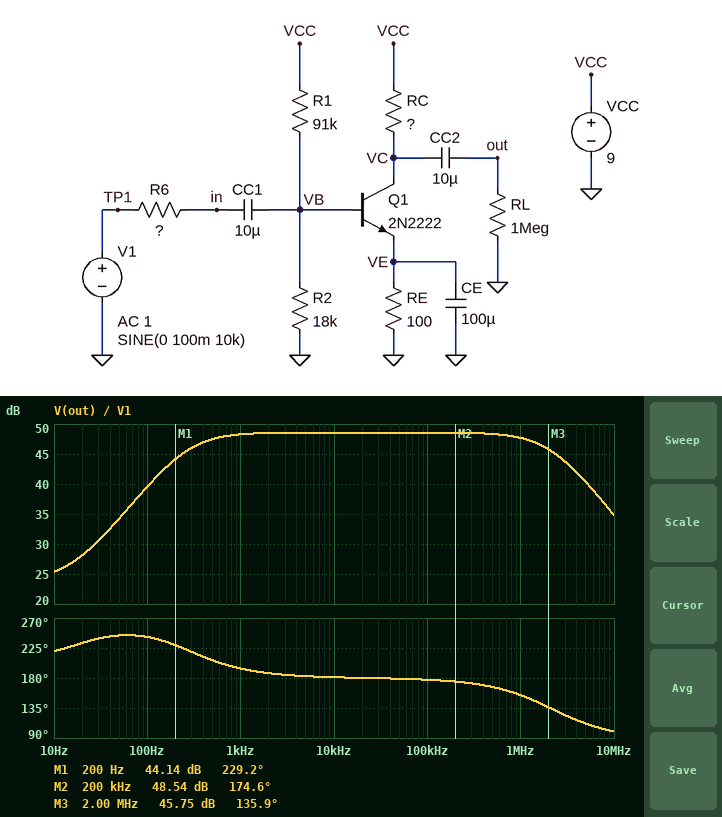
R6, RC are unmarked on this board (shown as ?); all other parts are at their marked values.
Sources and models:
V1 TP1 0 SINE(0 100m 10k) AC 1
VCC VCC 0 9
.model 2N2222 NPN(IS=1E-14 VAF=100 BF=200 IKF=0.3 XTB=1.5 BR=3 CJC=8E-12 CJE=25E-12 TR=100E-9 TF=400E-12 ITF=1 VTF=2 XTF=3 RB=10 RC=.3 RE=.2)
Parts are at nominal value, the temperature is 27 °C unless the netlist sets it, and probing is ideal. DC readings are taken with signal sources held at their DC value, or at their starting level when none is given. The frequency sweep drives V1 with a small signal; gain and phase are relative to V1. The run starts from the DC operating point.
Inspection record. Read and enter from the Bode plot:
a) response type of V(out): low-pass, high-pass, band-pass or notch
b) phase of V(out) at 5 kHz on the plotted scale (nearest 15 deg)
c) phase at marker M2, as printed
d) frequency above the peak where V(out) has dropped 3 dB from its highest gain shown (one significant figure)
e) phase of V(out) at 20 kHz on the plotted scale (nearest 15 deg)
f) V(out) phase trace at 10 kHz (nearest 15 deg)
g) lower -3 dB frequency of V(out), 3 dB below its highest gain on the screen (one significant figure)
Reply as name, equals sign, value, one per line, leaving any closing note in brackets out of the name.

response type of V(out): low-pass, high-pass, band-pass or notch = band-pass
phase of V(out) at 5 kHz on the plotted scale = 180 deg
phase at marker M2, as printed = 174.6 deg
frequency above the peak where V(out) has dropped 3 dB from its highest gain shown = 2 MHz
phase of V(out) at 20 kHz on the plotted scale = 180 deg
V(out) phase trace at 10 kHz = 180 deg
lower -3 dB frequency of V(out), 3 dB below its highest gain on the screen = 300 Hz
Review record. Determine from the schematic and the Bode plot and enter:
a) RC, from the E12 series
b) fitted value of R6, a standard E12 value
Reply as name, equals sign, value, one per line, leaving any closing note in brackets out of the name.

RC, from the E12 series = 1.8 kΩ
fitted value of R6, a standard E12 value = 15 Ω
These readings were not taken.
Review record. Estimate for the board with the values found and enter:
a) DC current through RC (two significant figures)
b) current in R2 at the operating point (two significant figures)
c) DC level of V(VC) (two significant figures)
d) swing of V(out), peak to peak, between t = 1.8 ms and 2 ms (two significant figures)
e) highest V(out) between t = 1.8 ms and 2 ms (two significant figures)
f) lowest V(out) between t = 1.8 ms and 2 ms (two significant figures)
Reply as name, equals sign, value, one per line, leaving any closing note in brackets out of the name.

DC current through RC = 4.5 mA
current in R2 at the operating point = 64 µA
DC level of V(VC) = 950 mV
swing of V(out), peak to peak, between t = 1.8 ms and 2 ms = 8.5 V
highest V(out) between t = 1.8 ms and 2 ms = 8.0 V
lowest V(out) between t = 1.8 ms and 2 ms = -510 mV
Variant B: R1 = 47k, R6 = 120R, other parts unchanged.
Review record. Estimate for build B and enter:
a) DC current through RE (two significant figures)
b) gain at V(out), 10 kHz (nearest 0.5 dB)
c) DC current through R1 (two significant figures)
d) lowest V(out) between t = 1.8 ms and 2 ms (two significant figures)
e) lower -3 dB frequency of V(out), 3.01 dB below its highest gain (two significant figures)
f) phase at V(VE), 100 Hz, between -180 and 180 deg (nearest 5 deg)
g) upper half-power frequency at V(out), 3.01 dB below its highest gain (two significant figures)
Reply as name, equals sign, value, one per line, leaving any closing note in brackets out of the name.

DC current through RE = 4.8 mA
gain at V(out), 10 kHz = 6.5 dB
DC current through R1 = 170 µA
lowest V(out) between t = 1.8 ms and 2 ms = -74 mV
lower -3 dB frequency of V(out), 3.01 dB below its highest gain = 120 Hz
phase at V(VE), 100 Hz, between -180 and 180 deg = -30 deg
upper half-power frequency at V(out), 3.01 dB below its highest gain = 590 kHz
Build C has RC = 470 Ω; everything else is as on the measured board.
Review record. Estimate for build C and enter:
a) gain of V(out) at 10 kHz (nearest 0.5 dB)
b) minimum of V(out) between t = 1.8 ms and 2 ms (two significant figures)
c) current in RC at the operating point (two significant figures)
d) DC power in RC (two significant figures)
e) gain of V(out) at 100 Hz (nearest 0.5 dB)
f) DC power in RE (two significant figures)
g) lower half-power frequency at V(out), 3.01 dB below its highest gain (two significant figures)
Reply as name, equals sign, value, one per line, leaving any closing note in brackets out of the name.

gain of V(out) at 10 kHz = 37.5 dB
minimum of V(out) between t = 1.8 ms and 2 ms = -6.3 V
current in RC at the operating point = 4.6 mA
DC power in RC = 9.9 mW
gain of V(out) at 100 Hz = 28.0 dB
DC power in RE = 2.1 mW
lower half-power frequency at V(out), 3.01 dB below its highest gain = 290 Hz
